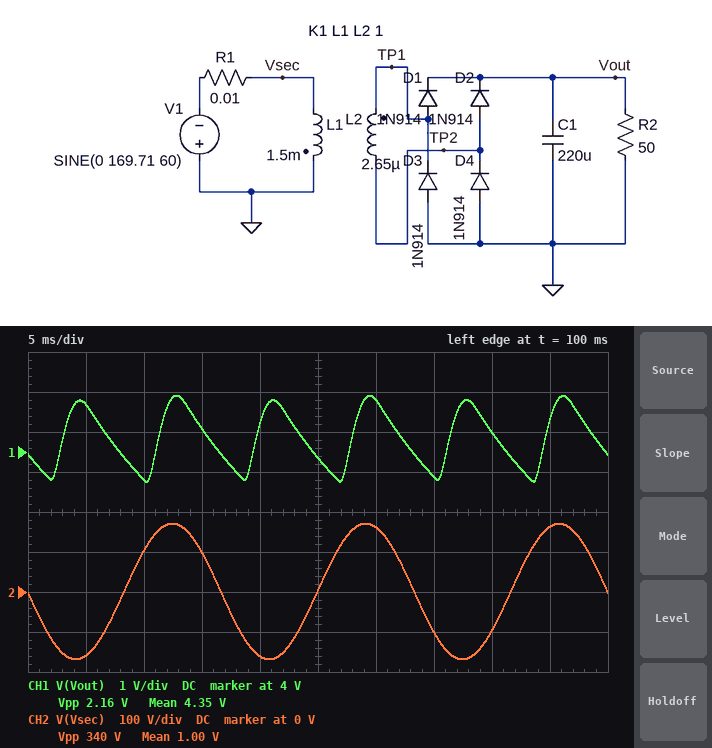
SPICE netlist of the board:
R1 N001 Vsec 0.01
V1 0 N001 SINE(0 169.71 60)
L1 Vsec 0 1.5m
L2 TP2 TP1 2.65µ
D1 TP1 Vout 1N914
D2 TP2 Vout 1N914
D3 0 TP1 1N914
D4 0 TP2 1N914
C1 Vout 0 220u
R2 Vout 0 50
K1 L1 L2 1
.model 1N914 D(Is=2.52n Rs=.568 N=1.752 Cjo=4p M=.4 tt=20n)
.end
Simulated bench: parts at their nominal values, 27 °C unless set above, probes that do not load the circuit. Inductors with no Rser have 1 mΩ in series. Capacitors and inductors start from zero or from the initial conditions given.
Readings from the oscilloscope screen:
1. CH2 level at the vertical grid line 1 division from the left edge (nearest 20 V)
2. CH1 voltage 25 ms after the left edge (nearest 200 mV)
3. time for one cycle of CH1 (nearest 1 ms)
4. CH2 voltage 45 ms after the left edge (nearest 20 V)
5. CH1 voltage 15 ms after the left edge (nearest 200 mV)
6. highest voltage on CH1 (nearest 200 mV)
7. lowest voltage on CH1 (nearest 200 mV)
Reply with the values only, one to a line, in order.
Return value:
-160 V
3.8 V
8 ms
160 V
4.6 V
5.4 V
3.2 V
